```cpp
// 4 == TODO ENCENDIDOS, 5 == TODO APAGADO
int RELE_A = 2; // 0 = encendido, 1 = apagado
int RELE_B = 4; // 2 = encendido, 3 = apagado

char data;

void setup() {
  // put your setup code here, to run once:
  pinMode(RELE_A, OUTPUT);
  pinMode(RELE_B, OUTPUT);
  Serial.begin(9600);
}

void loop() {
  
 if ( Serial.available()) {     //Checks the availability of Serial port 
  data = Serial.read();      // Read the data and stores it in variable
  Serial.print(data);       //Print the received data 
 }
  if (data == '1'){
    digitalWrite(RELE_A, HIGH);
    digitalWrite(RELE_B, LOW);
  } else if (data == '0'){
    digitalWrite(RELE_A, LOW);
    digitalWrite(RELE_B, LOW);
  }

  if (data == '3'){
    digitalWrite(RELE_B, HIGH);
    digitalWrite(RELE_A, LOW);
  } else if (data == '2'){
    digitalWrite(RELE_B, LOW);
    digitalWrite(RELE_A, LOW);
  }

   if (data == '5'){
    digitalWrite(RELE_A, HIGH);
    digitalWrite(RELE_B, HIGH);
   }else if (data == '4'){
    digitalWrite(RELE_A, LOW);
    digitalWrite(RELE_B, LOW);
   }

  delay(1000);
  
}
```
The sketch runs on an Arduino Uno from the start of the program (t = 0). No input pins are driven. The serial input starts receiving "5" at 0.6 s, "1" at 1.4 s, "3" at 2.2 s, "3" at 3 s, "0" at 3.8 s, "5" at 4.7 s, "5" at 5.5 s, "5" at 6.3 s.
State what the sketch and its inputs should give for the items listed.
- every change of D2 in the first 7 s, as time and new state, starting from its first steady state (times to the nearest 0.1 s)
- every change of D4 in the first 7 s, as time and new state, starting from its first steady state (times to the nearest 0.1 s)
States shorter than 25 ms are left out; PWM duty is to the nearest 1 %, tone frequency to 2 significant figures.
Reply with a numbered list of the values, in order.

1. 0 s low; 1 s high; 3 s low; 6 s high
2. 0 s low; 1 s high; 2 s low; 3 s high; 5 s low; 6 s high
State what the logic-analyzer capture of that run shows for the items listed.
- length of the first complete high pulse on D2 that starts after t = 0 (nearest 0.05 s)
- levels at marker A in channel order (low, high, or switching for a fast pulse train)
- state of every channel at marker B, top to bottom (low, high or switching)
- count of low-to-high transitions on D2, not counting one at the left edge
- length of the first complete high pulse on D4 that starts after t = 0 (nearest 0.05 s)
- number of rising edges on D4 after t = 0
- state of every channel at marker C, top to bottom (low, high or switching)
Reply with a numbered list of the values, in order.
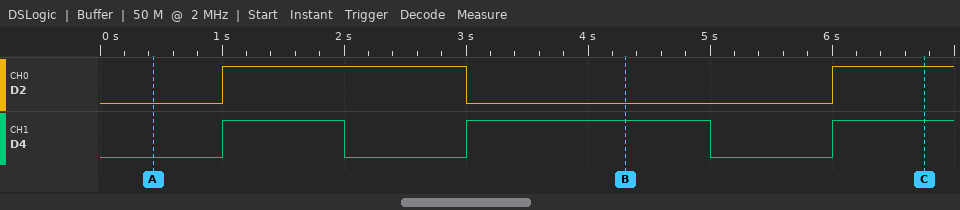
1. 2.00 s
2. D2 low, D4 low
3. D2 low, D4 high
4. 2
5. 1.00 s
6. 3
7. D2 high, D4 high
